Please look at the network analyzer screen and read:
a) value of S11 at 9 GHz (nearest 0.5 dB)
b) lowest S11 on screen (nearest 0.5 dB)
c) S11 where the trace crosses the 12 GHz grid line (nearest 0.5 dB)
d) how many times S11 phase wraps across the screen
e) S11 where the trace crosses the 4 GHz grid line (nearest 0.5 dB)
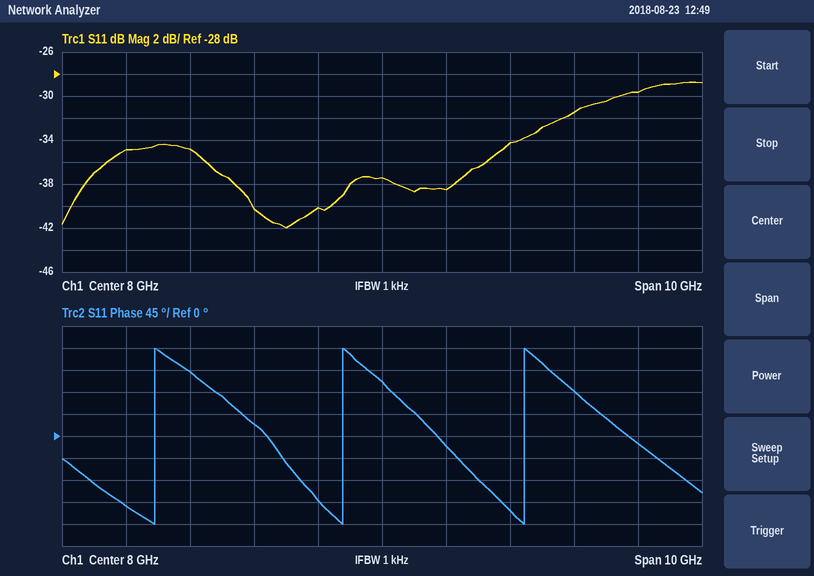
-38.5 dB
-42.0 dB
-29.5 dB
3
-35.0 dB
